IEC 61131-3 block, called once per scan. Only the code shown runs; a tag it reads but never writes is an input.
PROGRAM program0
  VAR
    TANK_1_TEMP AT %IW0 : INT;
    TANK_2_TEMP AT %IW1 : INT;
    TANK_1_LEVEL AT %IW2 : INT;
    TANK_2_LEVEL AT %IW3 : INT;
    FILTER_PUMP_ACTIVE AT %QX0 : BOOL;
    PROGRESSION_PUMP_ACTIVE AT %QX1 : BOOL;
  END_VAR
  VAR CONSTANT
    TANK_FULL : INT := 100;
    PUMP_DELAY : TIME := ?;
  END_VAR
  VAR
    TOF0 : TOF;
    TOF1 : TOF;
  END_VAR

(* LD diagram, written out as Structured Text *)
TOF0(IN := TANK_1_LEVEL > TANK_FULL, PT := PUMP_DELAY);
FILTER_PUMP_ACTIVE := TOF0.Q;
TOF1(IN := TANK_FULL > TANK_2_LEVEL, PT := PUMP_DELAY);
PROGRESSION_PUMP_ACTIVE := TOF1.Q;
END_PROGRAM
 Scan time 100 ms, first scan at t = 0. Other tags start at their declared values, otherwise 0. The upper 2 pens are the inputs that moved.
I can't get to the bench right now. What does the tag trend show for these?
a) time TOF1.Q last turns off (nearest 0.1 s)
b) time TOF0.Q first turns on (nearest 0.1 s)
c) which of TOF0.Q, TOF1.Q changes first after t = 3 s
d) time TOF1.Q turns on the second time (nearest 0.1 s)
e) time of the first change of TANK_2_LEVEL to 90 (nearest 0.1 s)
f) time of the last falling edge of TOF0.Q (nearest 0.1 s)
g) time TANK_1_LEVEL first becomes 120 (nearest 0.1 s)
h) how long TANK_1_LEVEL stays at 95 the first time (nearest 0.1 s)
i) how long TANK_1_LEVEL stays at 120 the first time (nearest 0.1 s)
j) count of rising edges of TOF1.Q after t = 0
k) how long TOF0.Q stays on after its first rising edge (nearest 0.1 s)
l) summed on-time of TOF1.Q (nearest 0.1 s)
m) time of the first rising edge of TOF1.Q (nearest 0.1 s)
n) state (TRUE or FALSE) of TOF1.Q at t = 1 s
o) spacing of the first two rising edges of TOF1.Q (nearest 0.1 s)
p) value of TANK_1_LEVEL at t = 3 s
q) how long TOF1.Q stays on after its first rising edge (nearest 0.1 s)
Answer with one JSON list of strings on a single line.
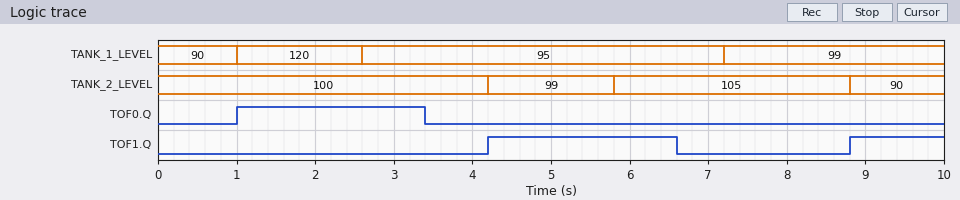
["6.6 s", "1.0 s", "TOF0.Q", "8.8 s", "8.8 s", "3.4 s", "1.0 s", "4.6 s", "1.6 s", "2", "2.4 s", "3.6 s", "4.2 s", "FALSE", "4.6 s", "95", "2.4 s"]
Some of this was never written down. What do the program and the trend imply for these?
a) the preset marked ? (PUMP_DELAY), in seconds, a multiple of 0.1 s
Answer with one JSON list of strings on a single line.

["0.8 s"]
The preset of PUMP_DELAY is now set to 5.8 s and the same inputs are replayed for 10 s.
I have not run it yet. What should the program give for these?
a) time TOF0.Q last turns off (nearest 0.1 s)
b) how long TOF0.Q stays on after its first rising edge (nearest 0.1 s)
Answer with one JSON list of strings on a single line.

["8.4 s", "7.4 s"]
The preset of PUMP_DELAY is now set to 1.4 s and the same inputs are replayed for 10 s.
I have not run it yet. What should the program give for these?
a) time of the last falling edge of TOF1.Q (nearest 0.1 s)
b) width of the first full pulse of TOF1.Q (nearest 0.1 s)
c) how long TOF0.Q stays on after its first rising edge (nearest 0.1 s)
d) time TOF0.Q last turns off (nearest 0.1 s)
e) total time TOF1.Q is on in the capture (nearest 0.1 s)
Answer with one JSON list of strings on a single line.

["7.2 s", "3.0 s", "3.0 s", "4.0 s", "4.2 s"]
